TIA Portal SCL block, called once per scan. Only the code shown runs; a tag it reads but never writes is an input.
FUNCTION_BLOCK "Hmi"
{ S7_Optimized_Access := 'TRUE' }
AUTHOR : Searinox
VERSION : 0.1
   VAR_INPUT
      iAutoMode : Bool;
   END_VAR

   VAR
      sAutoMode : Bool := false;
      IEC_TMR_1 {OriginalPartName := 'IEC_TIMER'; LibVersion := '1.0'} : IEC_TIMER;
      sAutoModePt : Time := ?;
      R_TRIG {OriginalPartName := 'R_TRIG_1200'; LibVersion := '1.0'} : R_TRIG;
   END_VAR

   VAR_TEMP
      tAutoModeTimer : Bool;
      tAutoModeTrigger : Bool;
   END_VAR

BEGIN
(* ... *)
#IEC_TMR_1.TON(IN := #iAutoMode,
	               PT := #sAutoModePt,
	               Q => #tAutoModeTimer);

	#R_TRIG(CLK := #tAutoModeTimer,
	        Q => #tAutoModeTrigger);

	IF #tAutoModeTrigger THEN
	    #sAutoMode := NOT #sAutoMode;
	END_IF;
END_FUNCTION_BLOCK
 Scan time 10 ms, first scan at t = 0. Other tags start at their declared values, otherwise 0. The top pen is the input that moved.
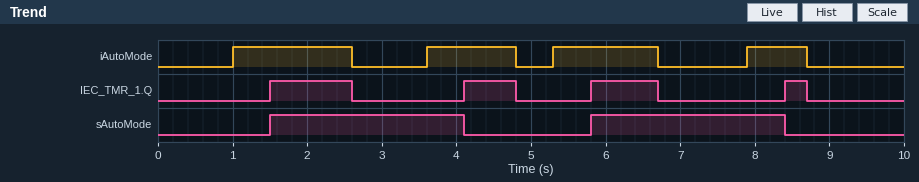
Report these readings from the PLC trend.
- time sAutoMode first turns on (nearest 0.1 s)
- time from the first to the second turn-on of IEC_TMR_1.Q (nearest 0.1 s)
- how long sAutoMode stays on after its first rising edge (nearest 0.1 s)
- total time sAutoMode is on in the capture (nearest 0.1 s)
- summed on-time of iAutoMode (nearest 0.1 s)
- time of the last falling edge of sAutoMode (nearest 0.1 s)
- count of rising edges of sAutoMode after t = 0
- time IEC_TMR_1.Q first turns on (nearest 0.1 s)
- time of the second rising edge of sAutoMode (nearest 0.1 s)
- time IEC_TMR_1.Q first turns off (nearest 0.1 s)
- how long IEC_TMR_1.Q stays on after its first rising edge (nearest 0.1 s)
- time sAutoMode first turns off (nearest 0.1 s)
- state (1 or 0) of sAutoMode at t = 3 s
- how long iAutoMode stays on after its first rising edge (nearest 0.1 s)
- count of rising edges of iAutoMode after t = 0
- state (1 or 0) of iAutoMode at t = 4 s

1.5 s
2.6 s
2.6 s
5.2 s
5.0 s
8.4 s
2
1.5 s
5.8 s
2.6 s
1.1 s
4.1 s
1
1.6 s
4
1
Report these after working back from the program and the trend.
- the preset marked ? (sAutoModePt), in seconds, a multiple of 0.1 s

0.5 s
